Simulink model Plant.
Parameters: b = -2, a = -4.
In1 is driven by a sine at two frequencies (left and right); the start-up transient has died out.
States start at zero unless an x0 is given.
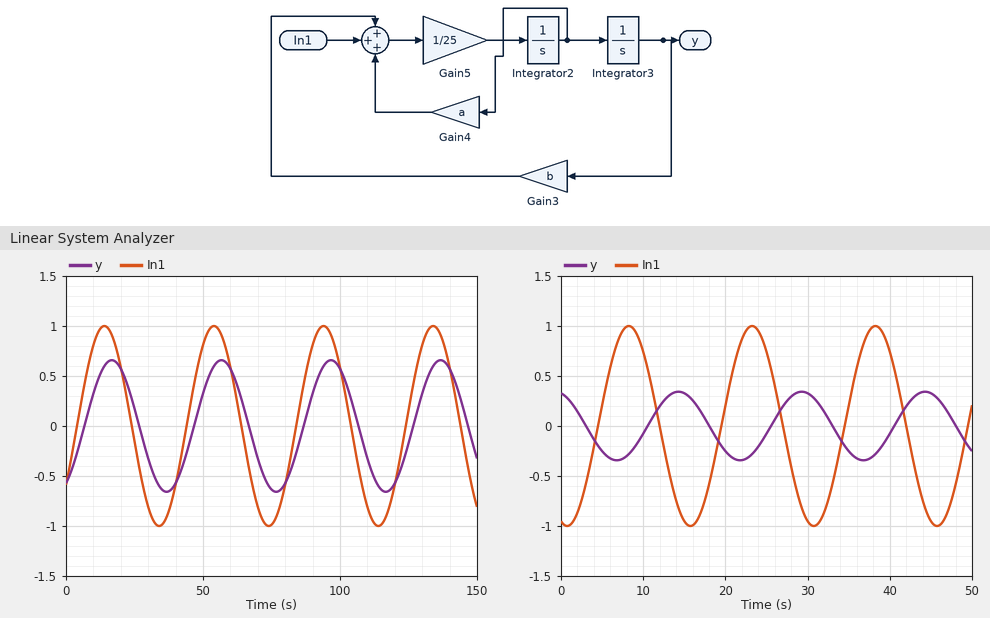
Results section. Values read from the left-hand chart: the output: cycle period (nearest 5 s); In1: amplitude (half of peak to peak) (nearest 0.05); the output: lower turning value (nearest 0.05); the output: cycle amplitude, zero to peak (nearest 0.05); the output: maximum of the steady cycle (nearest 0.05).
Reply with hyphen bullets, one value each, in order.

- 40 s
- 1.00
- -0.65
- 0.65
- 0.65
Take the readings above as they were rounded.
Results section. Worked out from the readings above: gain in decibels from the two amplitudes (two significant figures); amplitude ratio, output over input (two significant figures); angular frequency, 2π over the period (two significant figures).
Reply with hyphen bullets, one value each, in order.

- -3.7 dB
- 0.65
- 0.16 rad/s
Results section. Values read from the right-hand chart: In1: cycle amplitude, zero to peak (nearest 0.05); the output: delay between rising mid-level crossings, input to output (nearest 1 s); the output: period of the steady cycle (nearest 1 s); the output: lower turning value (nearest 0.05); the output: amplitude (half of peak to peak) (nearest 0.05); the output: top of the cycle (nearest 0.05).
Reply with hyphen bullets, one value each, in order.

- 1.00
- 6 s
- 15 s
- -0.35
- 0.35
- 0.35
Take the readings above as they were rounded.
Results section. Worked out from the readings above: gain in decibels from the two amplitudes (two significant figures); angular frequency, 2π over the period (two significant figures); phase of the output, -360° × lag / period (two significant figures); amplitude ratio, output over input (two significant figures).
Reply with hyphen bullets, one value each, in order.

- -9.1 dB
- 0.42 rad/s
- -140°
- 0.35
